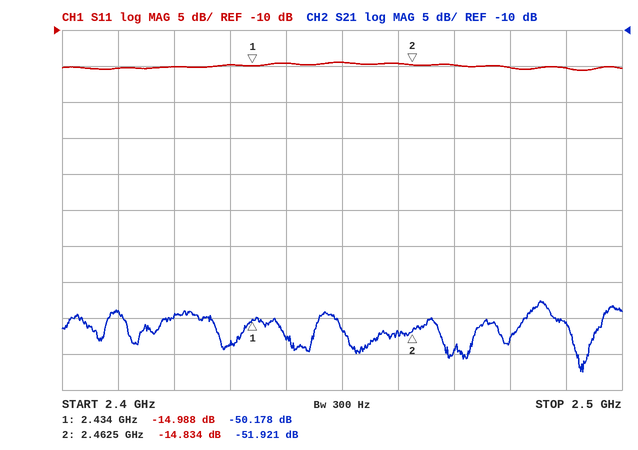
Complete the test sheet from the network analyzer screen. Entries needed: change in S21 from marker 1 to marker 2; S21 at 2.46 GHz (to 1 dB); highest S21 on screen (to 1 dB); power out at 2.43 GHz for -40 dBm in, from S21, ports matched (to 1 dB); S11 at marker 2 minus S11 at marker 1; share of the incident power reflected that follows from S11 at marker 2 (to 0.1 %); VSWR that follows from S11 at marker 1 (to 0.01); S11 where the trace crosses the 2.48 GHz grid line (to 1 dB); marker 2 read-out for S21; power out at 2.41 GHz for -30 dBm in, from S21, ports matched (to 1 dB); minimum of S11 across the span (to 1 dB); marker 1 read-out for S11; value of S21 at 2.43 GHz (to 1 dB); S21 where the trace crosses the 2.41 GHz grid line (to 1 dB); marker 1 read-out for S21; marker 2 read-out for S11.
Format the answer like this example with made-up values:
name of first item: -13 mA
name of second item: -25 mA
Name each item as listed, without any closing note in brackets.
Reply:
change in S21 from marker 1 to marker 2: -1.743 dB
S21 at 2.46 GHz: -52 dB
highest S21 on screen: -48 dB
power out at 2.43 GHz for -40 dBm in, from S21, ports matched: -94 dBm
S11 at marker 2 minus S11 at marker 1: 0.154 dB
share of the incident power reflected that follows from S11 at marker 2: 3.3 %
VSWR that follows from S11 at marker 1: 1.43
S11 where the trace crosses the 2.48 GHz grid line: -15 dB
marker 2 read-out for S21: -51.921 dB
power out at 2.41 GHz for -30 dBm in, from S21, ports matched: -79 dBm
minimum of S11 across the span: -16 dB
marker 1 read-out for S11: -14.988 dB
value of S21 at 2.43 GHz: -54 dB
S21 where the trace crosses the 2.41 GHz grid line: -49 dB
marker 1 read-out for S21: -50.178 dB
marker 2 read-out for S11: -14.834 dB
